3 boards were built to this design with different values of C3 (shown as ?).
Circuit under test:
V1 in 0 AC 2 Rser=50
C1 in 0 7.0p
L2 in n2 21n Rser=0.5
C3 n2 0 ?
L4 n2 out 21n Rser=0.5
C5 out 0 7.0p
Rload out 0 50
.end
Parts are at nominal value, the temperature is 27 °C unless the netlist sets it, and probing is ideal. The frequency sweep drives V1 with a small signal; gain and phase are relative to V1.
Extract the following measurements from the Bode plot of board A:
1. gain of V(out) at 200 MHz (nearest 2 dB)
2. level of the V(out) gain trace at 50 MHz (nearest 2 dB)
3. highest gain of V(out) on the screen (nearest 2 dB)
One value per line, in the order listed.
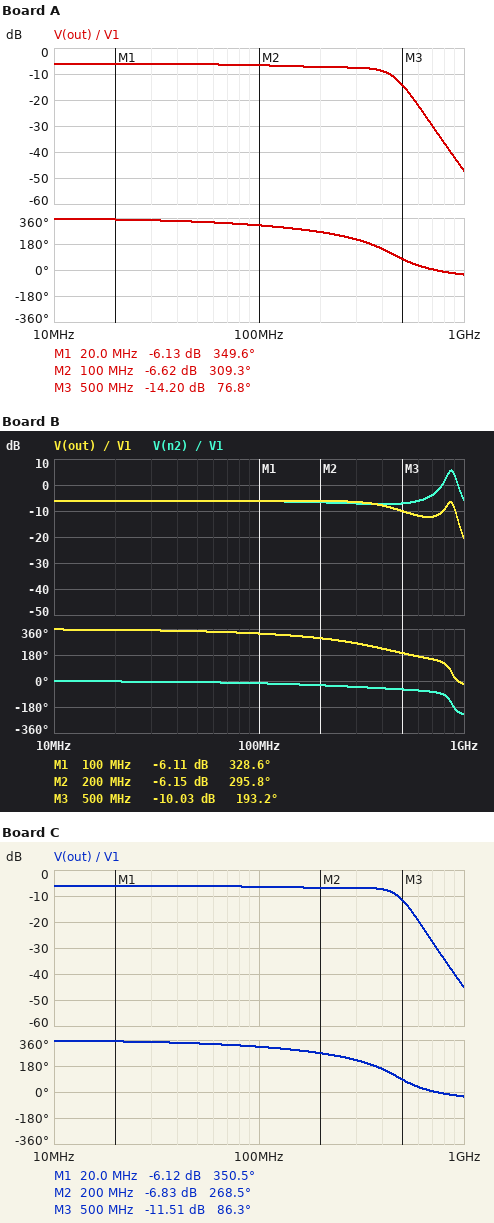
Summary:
-8 dB
-6 dB
-6 dB
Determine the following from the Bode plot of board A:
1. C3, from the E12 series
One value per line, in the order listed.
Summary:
27 pF
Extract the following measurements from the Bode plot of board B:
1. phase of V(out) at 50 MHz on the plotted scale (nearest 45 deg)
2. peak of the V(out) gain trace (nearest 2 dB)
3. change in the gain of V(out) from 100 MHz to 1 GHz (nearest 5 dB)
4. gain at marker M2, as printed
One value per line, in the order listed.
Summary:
360 deg
-6 dB
-15 dB
-6.15 dB
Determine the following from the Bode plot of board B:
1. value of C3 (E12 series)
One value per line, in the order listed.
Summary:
3.9 pF
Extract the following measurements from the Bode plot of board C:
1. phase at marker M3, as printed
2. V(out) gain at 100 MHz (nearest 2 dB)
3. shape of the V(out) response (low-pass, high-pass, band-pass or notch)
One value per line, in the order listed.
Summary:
86.3 deg
-6 dB
low-pass
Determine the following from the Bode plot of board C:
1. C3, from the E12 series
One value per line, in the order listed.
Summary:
22 pF
